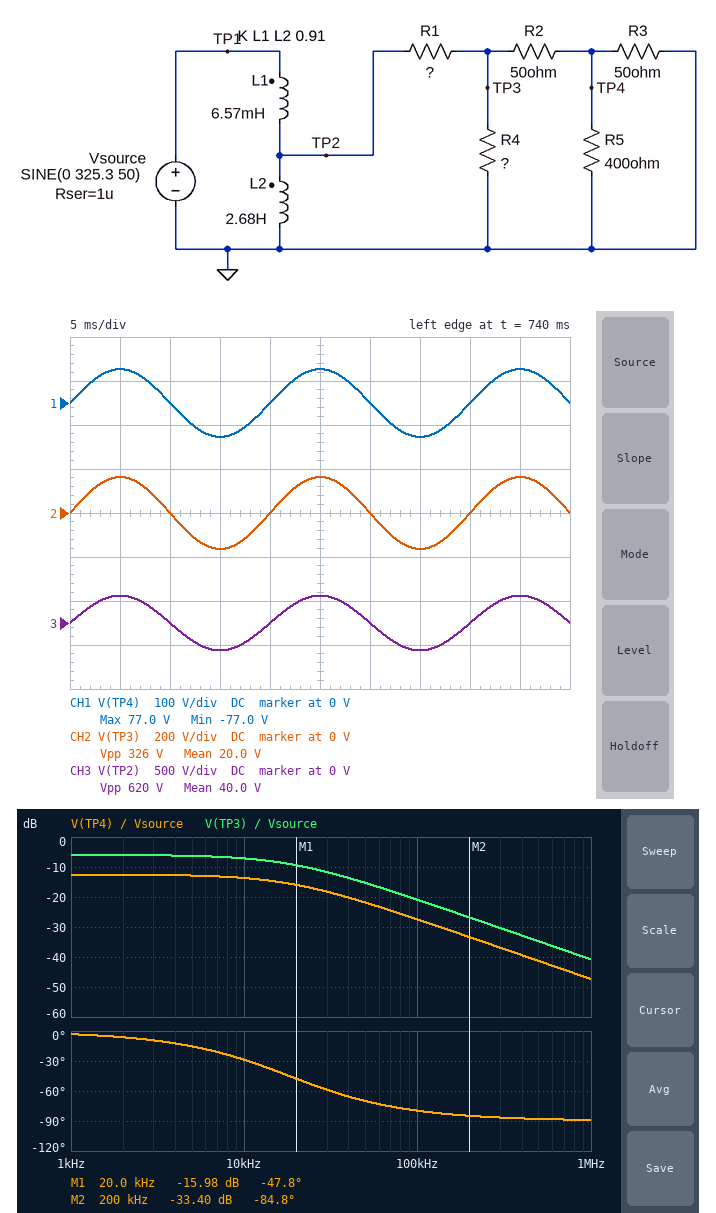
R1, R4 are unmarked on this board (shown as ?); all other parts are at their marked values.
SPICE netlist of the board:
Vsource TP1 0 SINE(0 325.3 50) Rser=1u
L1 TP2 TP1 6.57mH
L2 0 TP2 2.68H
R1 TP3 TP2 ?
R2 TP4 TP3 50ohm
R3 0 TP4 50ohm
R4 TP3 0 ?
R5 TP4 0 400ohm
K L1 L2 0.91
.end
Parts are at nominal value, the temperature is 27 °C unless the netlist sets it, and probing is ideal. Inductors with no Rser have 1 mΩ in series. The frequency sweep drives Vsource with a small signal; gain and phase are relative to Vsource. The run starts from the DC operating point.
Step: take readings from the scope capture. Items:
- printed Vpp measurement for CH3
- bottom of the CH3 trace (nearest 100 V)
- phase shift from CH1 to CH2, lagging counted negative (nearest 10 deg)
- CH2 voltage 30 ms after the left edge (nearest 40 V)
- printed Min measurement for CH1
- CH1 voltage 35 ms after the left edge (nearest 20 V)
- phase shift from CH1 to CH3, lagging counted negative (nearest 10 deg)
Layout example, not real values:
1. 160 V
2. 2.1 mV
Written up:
1. 620 V
2. -300 V
3. 0 deg
4. 0 V
5. -77.0 V
6. -80 V
7. 0 deg
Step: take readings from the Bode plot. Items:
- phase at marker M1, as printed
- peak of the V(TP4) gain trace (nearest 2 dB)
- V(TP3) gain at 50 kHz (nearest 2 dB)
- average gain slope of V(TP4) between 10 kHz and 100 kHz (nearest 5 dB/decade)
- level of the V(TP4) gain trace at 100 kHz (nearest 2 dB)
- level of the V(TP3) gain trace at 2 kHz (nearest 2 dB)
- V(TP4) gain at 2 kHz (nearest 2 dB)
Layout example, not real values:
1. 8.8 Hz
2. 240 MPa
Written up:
1. -47.8 deg
2. -12 dB
3. -16 dB
4. -15 dB/decade
5. -28 dB
6. -6 dB
7. -12 dB
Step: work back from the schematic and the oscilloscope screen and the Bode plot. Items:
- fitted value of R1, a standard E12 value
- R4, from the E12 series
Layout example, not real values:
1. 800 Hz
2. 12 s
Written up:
1. 56 Ω
2. 180 Ω
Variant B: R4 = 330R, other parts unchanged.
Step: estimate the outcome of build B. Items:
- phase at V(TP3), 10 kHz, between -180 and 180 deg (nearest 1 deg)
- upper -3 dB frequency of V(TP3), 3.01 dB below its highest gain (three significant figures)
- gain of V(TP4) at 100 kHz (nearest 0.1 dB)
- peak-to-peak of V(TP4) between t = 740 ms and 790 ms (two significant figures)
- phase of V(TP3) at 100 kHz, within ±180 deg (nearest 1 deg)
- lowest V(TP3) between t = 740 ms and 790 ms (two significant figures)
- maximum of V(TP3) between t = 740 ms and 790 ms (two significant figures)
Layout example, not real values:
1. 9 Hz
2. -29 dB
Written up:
1. -27 deg
2. 19.9 kHz
3. -26.0 dB
4. 170 V
5. -79 deg
6. -180 V
7. 180 V
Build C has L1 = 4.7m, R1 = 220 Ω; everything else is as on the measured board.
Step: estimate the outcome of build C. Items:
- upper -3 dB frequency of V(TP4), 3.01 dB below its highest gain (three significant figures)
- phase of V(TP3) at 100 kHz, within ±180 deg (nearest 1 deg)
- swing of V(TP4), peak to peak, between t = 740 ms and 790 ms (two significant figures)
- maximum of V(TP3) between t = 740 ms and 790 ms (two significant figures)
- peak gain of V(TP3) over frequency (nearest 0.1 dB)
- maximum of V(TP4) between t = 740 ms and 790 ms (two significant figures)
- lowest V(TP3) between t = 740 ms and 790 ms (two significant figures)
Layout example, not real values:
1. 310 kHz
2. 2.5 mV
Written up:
1. 59.9 kHz
2. -59 deg
3. 65 V
4. 69 V
5. -13.5 dB
6. 32 V
7. -69 V
